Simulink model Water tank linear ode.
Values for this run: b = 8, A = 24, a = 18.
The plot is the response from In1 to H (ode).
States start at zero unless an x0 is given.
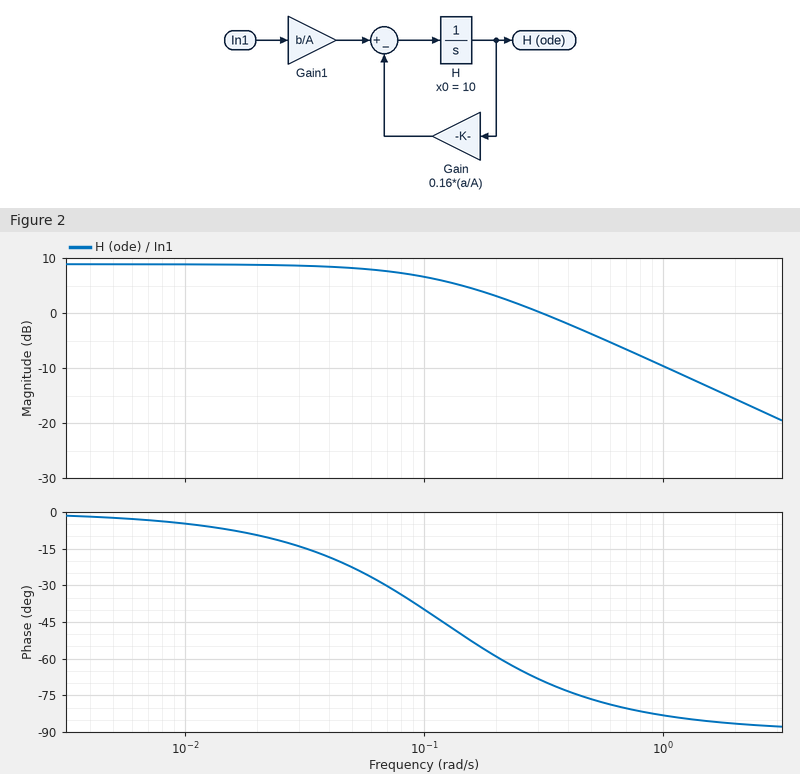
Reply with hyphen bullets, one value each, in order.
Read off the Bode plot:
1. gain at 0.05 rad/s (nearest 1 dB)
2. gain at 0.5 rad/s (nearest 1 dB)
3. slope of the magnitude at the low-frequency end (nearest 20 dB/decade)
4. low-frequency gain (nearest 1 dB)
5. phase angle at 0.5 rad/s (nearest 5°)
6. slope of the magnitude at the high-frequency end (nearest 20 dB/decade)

- 8 dB
- -4 dB
- 0 dB/decade
- 9 dB
- -75°
- -20 dB/decade
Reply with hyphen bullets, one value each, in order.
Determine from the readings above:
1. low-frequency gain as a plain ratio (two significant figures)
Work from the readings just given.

- 2.8
